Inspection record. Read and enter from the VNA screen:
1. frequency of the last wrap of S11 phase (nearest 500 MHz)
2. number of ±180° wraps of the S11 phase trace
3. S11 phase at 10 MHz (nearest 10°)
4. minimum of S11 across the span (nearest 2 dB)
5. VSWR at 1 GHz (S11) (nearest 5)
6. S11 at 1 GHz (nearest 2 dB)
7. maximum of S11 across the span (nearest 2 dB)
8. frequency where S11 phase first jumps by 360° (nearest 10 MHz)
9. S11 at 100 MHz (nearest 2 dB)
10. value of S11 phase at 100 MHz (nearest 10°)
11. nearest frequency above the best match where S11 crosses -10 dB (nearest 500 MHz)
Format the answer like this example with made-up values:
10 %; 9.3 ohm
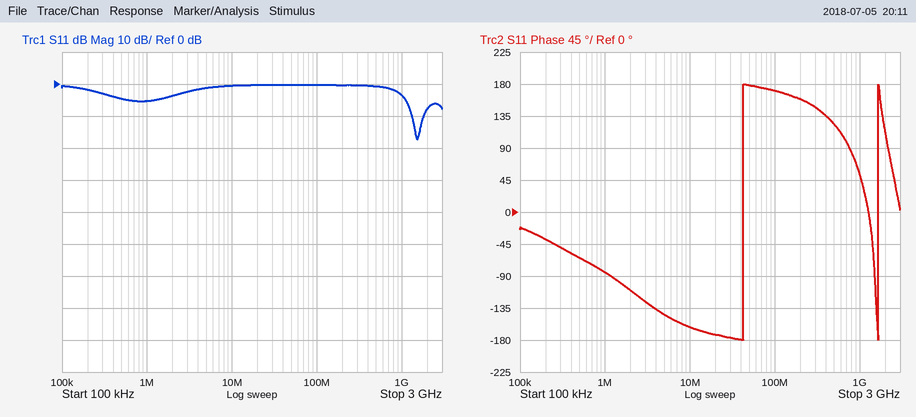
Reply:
1.5 GHz; 2; -160°; -18 dB; 5; -4 dB; 0 dB; 40 MHz; 0 dB; 170°; 2.0 GHz
